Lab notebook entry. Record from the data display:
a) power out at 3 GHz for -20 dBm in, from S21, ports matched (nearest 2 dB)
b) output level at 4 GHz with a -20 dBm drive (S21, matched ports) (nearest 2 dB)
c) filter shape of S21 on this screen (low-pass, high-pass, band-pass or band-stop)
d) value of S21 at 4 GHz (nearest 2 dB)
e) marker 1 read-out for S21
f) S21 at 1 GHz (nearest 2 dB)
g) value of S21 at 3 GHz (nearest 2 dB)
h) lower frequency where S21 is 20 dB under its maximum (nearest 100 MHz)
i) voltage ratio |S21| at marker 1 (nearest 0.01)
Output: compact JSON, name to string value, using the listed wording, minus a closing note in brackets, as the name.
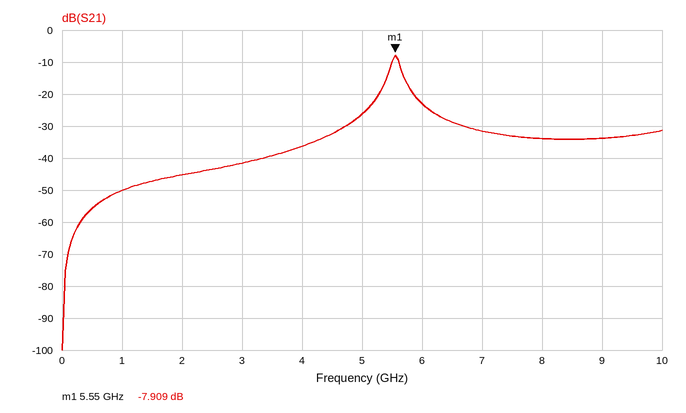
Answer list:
{"power out at 3 GHz for -20 dBm in, from S21, ports matched": "-62 dBm", "output level at 4 GHz with a -20 dBm drive (S21, matched ports)": "-56 dBm", "filter shape of S21 on this screen": "band-pass", "value of S21 at 4 GHz": "-36 dB", "marker 1 read-out for S21": "-7.909 dB", "S21 at 1 GHz": "-50 dB", "value of S21 at 3 GHz": "-42 dB", "lower frequency where S21 is 20 dB under its maximum": "4.9 GHz", "voltage ratio |S21| at marker 1": "0.40"}
